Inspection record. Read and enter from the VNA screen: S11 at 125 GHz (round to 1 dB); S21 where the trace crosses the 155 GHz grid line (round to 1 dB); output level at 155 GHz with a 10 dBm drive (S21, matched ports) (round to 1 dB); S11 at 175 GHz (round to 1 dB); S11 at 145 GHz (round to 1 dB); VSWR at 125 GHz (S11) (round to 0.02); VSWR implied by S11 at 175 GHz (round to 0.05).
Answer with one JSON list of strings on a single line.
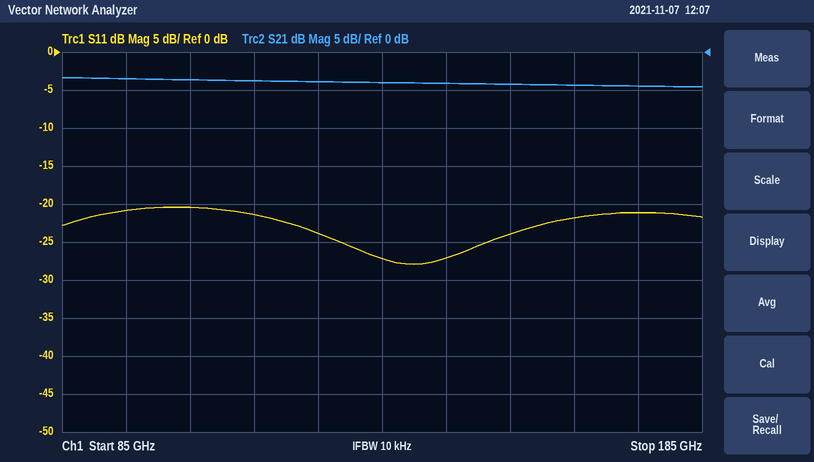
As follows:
["-24 dB", "-4 dB", "6 dBm", "-21 dB", "-27 dB", "1.14", "1.20"]
